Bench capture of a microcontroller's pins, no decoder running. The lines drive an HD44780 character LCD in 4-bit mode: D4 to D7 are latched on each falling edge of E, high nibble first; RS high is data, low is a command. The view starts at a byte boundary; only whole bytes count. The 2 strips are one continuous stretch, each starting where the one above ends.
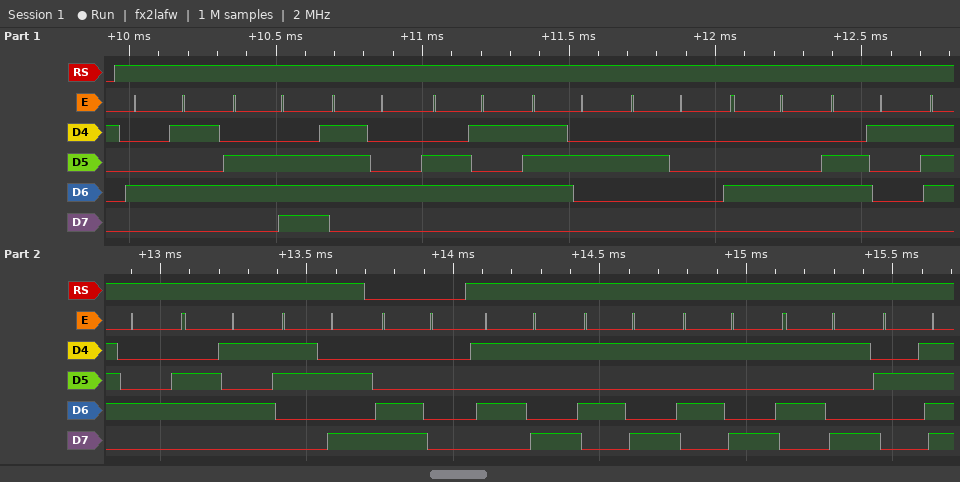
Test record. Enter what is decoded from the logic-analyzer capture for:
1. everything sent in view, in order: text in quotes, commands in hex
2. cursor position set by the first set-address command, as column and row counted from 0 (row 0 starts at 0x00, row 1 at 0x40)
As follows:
"Enter Date:" 0xC0 "YYYY/"
column 0, row 1
